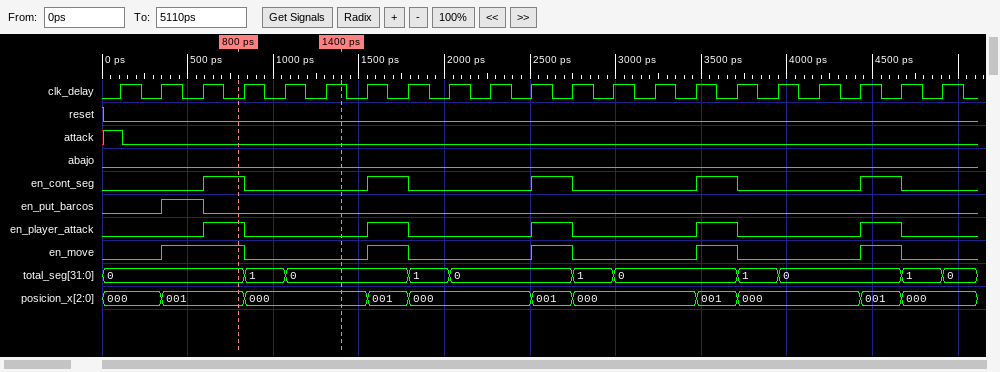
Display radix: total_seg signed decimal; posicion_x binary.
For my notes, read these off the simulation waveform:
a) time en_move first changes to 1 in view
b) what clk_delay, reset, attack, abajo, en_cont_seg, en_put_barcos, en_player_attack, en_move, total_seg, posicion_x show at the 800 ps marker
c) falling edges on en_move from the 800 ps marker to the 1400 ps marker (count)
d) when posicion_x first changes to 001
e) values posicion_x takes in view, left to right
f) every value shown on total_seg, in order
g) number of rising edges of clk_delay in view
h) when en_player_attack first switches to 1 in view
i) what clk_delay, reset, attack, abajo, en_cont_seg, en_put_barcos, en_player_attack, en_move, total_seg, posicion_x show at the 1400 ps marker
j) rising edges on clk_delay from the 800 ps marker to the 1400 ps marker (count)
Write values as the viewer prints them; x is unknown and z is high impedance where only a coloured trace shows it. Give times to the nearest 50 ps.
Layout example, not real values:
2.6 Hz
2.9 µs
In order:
350 ps
clk_delay=0, reset=0, attack=0, abajo=0, en_cont_seg=1, en_put_barcos=0, en_player_attack=1, en_move=1, total_seg=0, posicion_x=001
1
350 ps
000, 001, 000, 001, 000, 001, 000, 001, 000, 001, 000
0, 1, 0, 1, 0, 1, 0, 1, 0, 1, 0
21
600 ps
clk_delay=1, reset=0, attack=0, abajo=0, en_cont_seg=0, en_put_barcos=0, en_player_attack=0, en_move=0, total_seg=0, posicion_x=000
3
